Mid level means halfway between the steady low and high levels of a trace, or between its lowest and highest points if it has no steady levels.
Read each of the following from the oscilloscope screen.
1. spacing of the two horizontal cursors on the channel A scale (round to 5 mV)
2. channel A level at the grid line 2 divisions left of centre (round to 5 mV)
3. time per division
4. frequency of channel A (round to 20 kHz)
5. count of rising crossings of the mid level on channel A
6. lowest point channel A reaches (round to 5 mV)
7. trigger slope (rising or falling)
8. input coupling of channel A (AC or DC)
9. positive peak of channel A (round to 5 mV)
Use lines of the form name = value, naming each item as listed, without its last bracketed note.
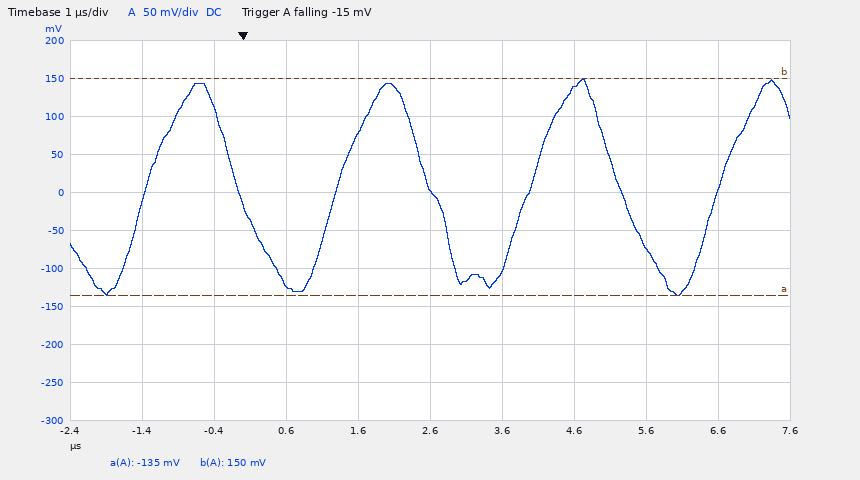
spacing of the two horizontal cursors on the channel A scale = 285 mV
channel A level at the grid line 2 divisions left of centre = -120 mV
time per division = 1 µs
frequency of channel A = 380 kHz
count of rising crossings of the mid level on channel A = 4
lowest point channel A reaches = -135 mV
trigger slope = falling
input coupling of channel A = DC
positive peak of channel A = 150 mV
